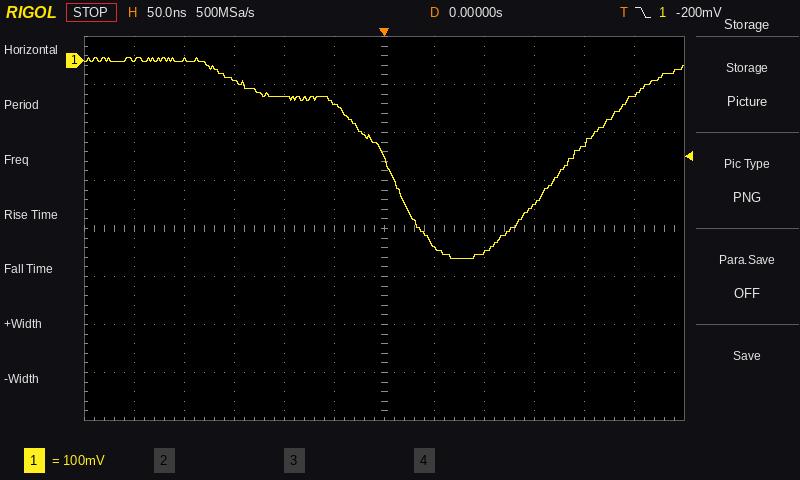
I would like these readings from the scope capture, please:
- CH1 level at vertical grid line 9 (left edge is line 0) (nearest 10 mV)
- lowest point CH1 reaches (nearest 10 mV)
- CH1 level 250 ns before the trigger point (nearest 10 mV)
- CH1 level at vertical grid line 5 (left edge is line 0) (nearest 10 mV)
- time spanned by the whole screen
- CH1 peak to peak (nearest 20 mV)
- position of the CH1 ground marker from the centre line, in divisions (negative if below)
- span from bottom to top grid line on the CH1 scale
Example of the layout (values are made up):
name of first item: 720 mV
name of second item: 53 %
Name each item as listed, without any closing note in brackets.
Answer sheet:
CH1 level at vertical grid line 9 (left edge is line 0): -300 mV
lowest point CH1 reaches: -410 mV
CH1 level 250 ns before the trigger point: 0 mV
CH1 level at vertical grid line 5 (left edge is line 0): -90 mV
time spanned by the whole screen: 600 ns
CH1 peak to peak: 420 mV
position of the CH1 ground marker from the centre line, in divisions: +3.5 div
span from bottom to top grid line on the CH1 scale: 800 mV
